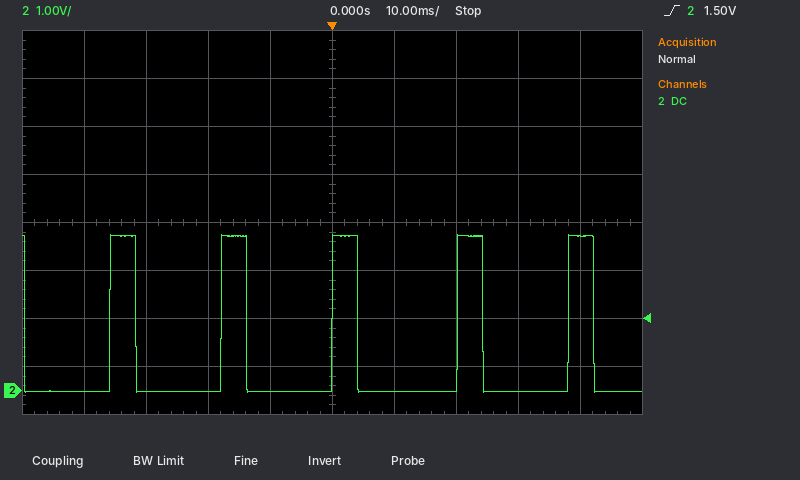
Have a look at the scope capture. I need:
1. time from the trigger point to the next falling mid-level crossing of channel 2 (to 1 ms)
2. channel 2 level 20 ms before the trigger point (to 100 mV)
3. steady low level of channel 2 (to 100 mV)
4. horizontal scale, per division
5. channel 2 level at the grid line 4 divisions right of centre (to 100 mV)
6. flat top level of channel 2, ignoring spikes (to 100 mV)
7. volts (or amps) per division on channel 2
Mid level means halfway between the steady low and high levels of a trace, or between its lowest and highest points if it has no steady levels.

4 ms
0.0 V
0.0 V
10 ms
3.2 V
3.2 V
1 V
